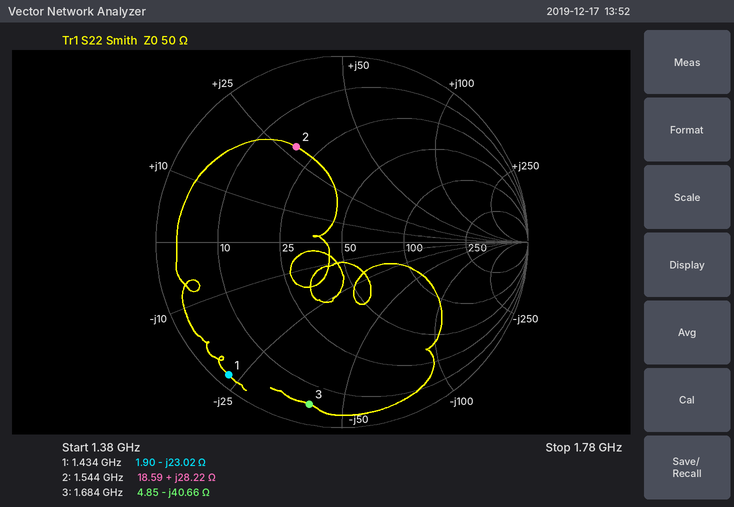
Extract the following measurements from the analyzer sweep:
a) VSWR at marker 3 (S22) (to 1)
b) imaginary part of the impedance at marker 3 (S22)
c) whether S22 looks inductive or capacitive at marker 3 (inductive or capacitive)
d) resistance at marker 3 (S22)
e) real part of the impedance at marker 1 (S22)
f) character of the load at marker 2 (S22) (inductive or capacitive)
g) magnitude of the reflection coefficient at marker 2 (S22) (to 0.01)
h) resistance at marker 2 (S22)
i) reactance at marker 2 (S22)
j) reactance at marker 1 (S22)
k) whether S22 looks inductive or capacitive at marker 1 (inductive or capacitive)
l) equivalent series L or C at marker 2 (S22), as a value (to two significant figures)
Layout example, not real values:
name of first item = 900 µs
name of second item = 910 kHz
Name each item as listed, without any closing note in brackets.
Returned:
VSWR at marker 3 (S22) = 17
imaginary part of the impedance at marker 3 = -40.66 Ω
whether S22 looks inductive or capacitive at marker 3 = capacitive
resistance at marker 3 = 4.85 Ω
real part of the impedance at marker 1 = 1.90 Ω
character of the load at marker 2 (S22) = inductive
magnitude of the reflection coefficient at marker 2 (S22) = 0.57
resistance at marker 2 = 18.59 Ω
reactance at marker 2 = +28.22 Ω
reactance at marker 1 = -23.02 Ω
whether S22 looks inductive or capacitive at marker 1 = capacitive
equivalent series L or C at marker 2 (S22), as a value = 2.9 nH
